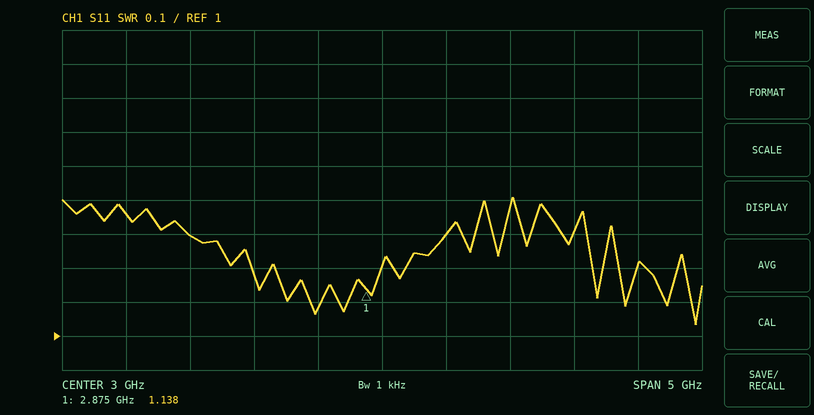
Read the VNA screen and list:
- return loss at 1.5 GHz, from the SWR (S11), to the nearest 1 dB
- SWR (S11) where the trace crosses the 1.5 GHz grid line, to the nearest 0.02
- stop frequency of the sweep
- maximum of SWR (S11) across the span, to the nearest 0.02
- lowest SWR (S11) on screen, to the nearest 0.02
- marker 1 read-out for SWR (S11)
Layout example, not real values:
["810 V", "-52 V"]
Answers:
["18 dB", "1.30", "5.5 GHz", "1.40", "1.04", "1.138"]
